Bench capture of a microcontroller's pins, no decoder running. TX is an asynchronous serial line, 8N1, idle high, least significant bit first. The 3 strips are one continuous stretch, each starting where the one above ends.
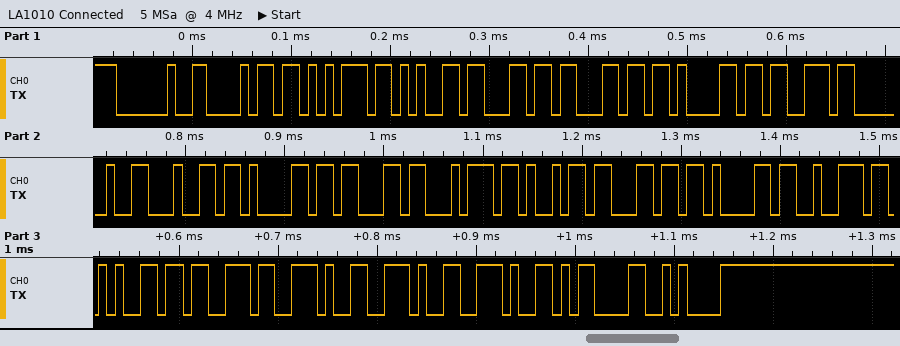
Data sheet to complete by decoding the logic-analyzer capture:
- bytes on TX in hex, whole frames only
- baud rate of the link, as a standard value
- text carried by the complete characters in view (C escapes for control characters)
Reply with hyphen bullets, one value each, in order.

- 20 68 75 65 6C 6C 61 73 20 64 61 63 74 69 6C 61 72 65 73 2E 2E 2E 0D 0A
- 115200 baud
- " huellas dactilares...\r\n"
